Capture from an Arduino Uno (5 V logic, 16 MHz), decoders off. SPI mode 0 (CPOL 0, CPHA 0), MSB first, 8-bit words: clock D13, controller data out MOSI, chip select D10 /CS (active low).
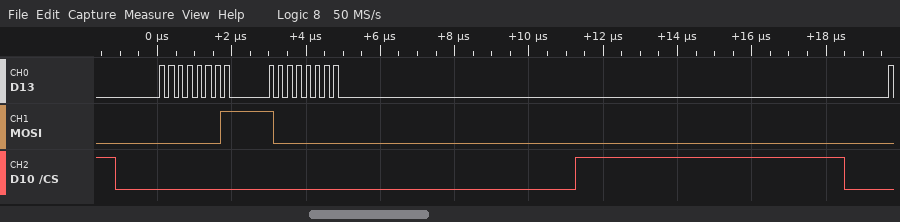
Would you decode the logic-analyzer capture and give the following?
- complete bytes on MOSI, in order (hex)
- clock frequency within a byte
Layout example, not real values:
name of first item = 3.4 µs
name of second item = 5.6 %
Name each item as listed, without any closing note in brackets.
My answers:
complete bytes on MOSI, in order = 01 80
clock frequency within a byte = 4 MHz
